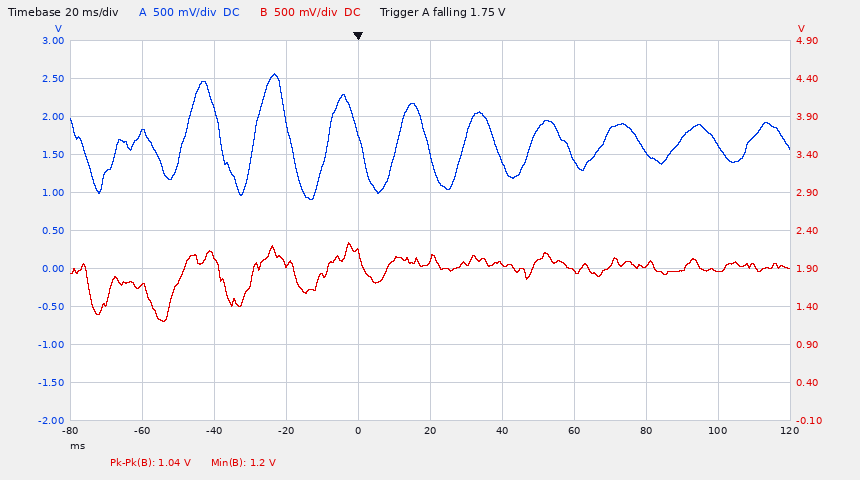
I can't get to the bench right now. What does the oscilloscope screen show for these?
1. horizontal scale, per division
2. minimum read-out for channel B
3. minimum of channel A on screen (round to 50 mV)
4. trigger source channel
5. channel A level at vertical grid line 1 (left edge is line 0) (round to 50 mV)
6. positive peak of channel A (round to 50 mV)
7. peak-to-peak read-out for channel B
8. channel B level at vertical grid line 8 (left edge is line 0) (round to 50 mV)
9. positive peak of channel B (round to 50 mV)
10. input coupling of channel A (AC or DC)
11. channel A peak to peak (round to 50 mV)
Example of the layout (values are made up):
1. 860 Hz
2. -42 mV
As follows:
1. 20 ms
2. 1.2 V
3. 900 mV
4. channel A
5. 1.80 V
6. 2.55 V
7. 1.04 V
8. 1.95 V
9. 2.25 V
10. DC
11. 1.65 V
